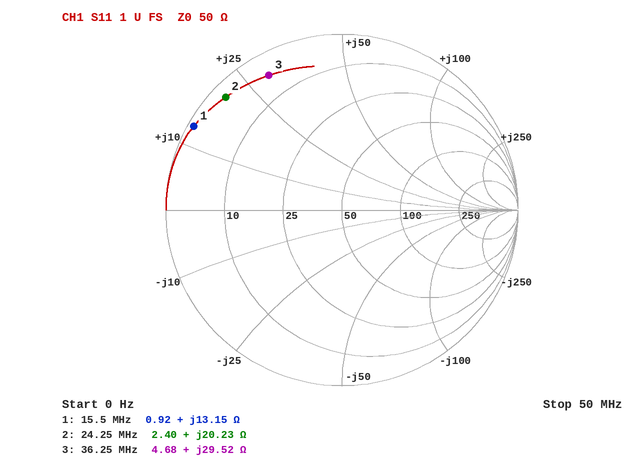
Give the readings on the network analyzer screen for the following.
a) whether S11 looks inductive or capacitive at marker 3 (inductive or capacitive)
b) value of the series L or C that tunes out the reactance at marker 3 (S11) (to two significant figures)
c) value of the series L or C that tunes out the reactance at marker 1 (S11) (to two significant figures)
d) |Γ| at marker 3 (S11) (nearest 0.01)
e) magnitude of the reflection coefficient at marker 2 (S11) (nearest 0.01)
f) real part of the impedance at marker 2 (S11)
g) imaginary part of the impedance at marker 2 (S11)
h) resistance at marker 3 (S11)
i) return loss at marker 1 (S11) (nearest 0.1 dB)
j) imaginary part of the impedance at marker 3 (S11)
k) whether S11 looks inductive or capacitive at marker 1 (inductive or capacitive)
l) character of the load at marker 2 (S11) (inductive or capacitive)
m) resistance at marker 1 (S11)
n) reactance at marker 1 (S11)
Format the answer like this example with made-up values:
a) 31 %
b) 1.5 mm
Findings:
a) inductive
b) 150 pF
c) 780 pF
d) 0.87
e) 0.92
f) 2.40 Ω
g) +20.23 Ω
h) 4.68 Ω
i) 0.3 dB
j) +29.52 Ω
k) inductive
l) inductive
m) 0.92 Ω
n) +13.15 Ω
